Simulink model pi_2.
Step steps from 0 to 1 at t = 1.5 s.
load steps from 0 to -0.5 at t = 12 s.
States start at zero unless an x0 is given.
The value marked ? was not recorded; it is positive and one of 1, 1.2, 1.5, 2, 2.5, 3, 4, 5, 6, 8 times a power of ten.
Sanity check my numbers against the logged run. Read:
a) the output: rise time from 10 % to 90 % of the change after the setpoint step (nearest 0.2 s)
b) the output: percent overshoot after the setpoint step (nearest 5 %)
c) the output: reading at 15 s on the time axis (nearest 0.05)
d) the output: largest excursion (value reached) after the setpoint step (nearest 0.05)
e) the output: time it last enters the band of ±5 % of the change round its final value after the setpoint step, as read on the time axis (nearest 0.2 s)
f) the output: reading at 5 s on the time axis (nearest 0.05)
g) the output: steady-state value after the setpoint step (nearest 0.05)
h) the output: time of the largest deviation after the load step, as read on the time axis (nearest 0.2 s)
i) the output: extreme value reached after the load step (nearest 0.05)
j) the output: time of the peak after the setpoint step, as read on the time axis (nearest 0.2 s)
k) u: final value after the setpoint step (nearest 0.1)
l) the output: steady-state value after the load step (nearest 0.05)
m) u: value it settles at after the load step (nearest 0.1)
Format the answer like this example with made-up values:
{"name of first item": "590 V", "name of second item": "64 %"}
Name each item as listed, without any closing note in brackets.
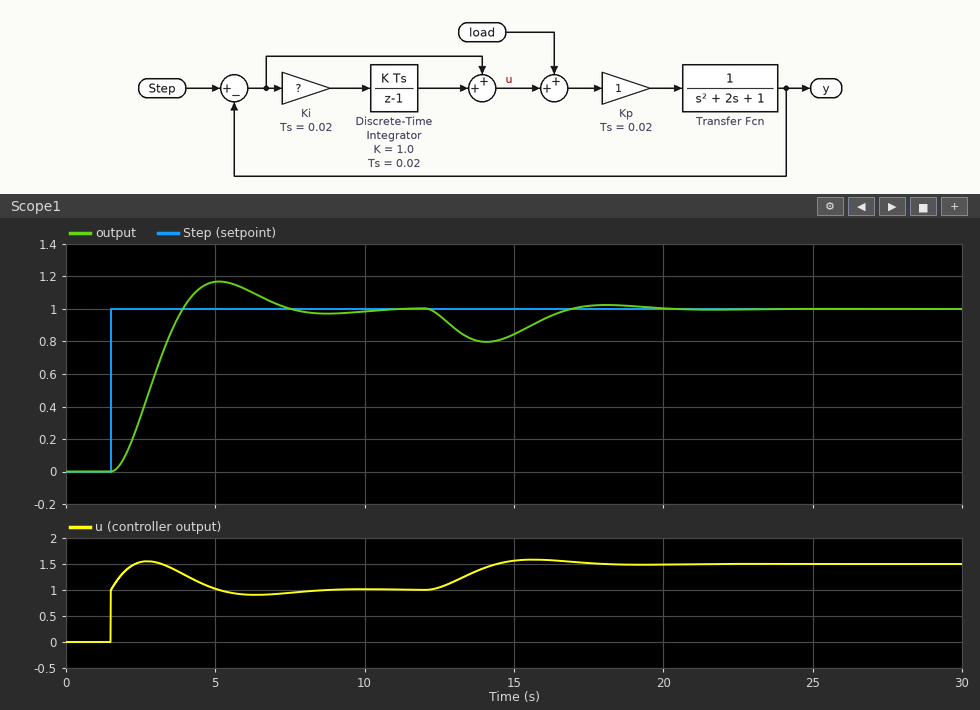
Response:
{"the output: rise time from 10 % to 90 % of the change after the setpoint step": "1.6 s", "the output: percent overshoot after the setpoint step": "15 %", "the output: reading at 15 s on the time axis": "0.85", "the output: largest excursion (value reached) after the setpoint step": "1.15", "the output: time it last enters the band of ±5 % of the change round its final value after the setpoint step, as read on the time axis": "6.8 s", "the output: reading at 5 s on the time axis": "1.15", "the output: steady-state value after the setpoint step": "1.00", "the output: time of the largest deviation after the load step, as read on the time axis": "14.0 s", "the output: extreme value reached after the load step": "0.80", "the output: time of the peak after the setpoint step, as read on the time axis": "5.2 s", "u: final value after the setpoint step": "1.0", "the output: steady-state value after the load step": "1.00", "u: value it settles at after the load step": "1.5"}
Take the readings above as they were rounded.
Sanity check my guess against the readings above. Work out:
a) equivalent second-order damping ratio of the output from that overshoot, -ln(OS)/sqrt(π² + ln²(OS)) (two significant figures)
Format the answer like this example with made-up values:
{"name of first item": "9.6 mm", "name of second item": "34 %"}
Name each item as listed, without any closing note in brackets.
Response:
{"equivalent second-order damping ratio of the output from that overshoot, -ln(OS)/sqrt(π² + ln²(OS))": "0.52"}
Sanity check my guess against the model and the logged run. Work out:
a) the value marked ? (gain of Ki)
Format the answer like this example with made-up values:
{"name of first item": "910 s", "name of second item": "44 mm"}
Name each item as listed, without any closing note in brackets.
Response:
{"the value marked ?": "1"}
